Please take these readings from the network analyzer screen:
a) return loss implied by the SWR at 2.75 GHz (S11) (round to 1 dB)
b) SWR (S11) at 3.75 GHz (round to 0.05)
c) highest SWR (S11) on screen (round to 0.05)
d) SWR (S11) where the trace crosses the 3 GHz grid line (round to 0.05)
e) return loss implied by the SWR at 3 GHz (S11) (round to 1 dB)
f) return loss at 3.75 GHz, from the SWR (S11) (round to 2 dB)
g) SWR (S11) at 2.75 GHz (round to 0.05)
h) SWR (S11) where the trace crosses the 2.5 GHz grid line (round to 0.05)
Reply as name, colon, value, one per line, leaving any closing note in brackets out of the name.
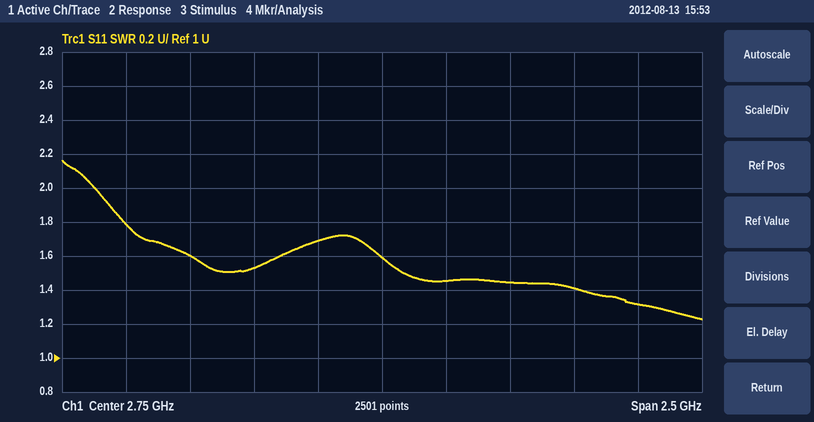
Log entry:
return loss implied by the SWR at 2.75 GHz (S11): 13 dB
SWR (S11) at 3.75 GHz: 1.30
highest SWR (S11) on screen: 2.15
SWR (S11) where the trace crosses the 3 GHz grid line: 1.45
return loss implied by the SWR at 3 GHz (S11): 15 dB
return loss at 3.75 GHz, from the SWR (S11): 18 dB
SWR (S11) at 2.75 GHz: 1.60
SWR (S11) where the trace crosses the 2.5 GHz grid line: 1.70
